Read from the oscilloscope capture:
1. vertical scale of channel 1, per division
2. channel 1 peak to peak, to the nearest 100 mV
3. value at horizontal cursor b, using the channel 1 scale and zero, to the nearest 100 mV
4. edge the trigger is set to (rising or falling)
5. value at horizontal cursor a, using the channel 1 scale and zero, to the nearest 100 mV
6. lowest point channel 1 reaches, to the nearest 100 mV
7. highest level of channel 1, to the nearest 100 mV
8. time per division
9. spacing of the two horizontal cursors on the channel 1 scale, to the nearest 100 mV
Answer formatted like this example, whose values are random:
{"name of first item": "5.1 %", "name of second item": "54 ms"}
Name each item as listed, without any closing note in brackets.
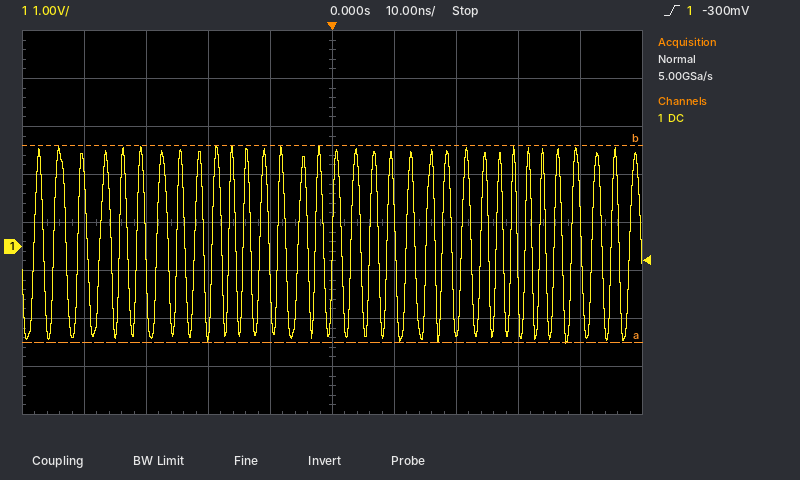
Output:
{"vertical scale of channel 1, per division": "1 V", "channel 1 peak to peak, to the nearest 100 mV": "4.1 V", "value at horizontal cursor b, using the channel 1 scale and zero, to the nearest 100 mV": "2.1 V", "edge the trigger is set to": "rising", "value at horizontal cursor a, using the channel 1 scale and zero, to the nearest 100 mV": "-2.0 V", "lowest point channel 1 reaches, to the nearest 100 mV": "-2.0 V", "highest level of channel 1, to the nearest 100 mV": "2.1 V", "time per division": "10 ns", "spacing of the two horizontal cursors on the channel 1 scale, to the nearest 100 mV": "4.1 V"}
